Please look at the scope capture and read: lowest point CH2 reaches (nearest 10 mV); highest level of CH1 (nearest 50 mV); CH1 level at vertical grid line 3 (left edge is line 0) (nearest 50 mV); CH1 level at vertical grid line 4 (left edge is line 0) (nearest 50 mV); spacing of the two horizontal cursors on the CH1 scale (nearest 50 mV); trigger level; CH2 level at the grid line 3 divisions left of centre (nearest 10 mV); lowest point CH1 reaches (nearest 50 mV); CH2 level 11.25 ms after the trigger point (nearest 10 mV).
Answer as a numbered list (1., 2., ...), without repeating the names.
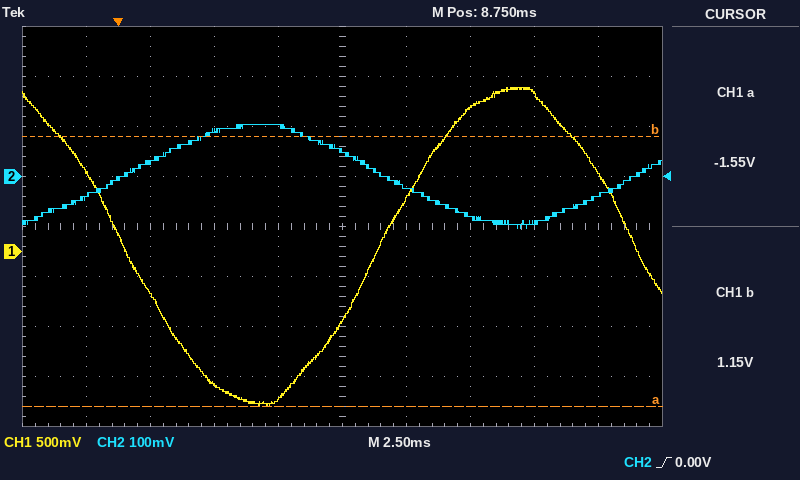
1. -100 mV
2. 1.65 V
3. -1.35 V
4. -1.45 V
5. 2.70 V
6. 0.00 V
7. 30 mV
8. -1.55 V
9. -20 mV
